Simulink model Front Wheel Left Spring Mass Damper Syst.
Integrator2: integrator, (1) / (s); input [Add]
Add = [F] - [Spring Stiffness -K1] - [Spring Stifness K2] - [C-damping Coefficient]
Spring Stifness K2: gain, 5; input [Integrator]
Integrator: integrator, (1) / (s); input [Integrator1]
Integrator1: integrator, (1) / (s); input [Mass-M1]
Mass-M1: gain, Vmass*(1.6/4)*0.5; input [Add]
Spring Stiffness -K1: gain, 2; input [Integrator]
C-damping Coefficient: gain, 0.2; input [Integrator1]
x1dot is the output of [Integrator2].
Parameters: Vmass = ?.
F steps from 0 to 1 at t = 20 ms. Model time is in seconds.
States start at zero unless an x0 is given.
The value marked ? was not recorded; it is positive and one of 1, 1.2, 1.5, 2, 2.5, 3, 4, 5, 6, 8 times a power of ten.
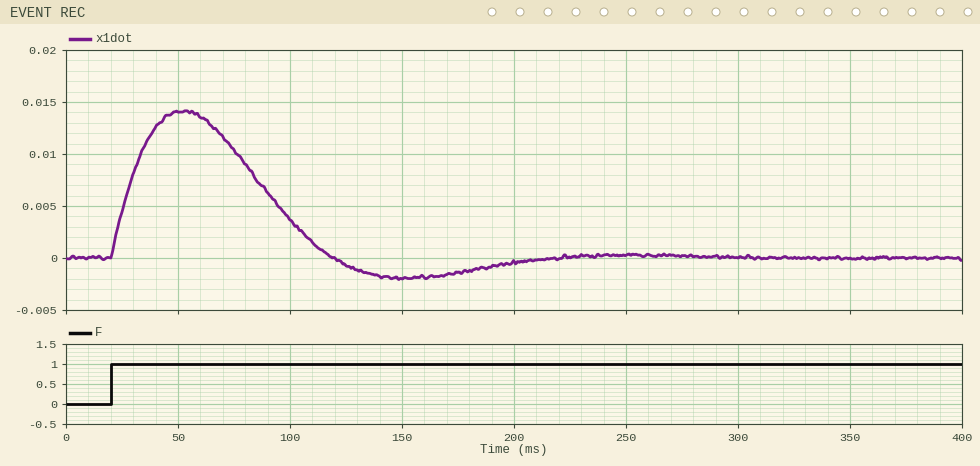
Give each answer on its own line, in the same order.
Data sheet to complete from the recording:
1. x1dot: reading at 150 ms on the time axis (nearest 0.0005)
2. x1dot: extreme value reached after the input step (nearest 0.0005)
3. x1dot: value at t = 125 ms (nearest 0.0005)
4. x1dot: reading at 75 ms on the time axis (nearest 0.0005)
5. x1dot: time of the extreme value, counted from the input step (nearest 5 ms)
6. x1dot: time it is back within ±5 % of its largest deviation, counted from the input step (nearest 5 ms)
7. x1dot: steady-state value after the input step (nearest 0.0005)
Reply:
-0.0020
0.0140
-0.0005
0.0105
30 ms
175 ms
0.0000
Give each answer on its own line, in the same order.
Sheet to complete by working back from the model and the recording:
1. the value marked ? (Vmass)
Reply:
1000
